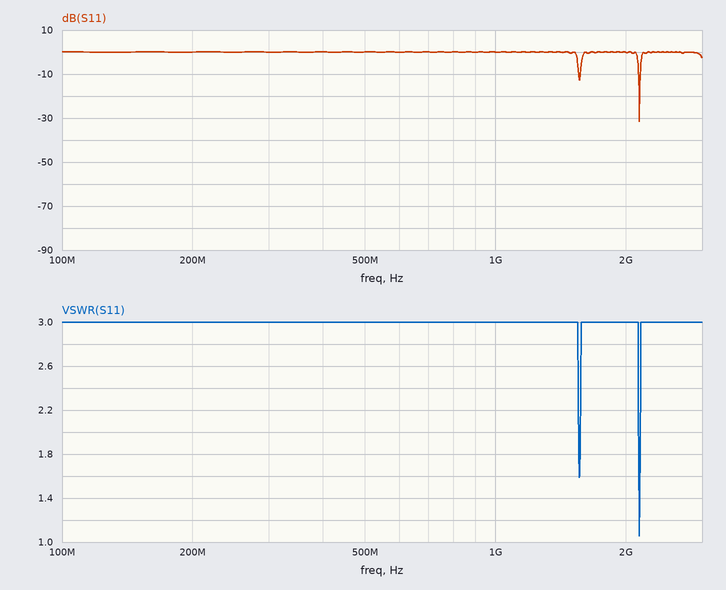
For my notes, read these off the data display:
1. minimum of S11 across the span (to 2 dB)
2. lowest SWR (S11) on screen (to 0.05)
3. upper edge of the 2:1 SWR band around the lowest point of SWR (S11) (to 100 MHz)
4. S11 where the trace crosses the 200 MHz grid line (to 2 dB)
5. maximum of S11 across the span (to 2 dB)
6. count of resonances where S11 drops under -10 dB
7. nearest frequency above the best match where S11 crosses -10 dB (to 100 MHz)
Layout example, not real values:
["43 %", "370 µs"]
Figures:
["-32 dB", "1.05", "2.2 GHz", "0 dB", "0 dB", "2", "2.2 GHz"]
